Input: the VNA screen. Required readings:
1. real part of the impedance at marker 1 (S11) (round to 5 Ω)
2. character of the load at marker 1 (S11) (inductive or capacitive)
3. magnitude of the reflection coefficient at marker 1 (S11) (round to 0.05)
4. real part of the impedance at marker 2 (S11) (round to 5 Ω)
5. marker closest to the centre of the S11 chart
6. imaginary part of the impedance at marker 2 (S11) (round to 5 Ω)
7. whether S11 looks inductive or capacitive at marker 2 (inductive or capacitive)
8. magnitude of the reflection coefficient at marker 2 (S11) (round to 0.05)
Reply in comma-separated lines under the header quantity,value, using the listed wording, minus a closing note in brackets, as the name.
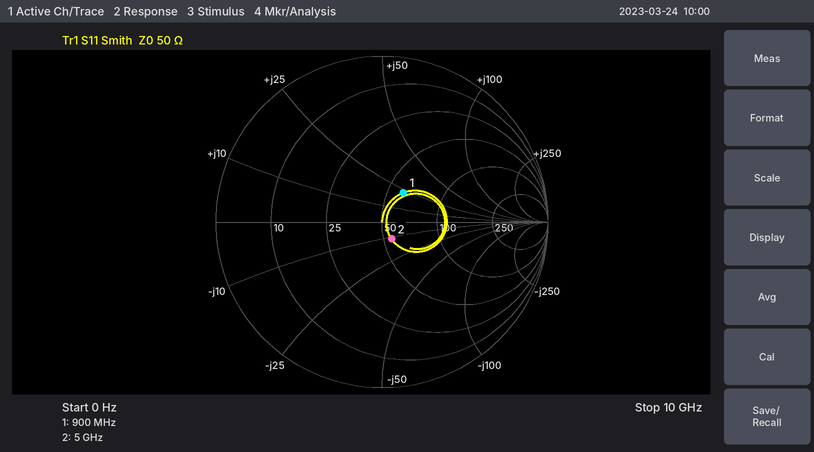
quantity,value
real part of the impedance at marker 1 (S11),60 Ω
character of the load at marker 1 (S11),inductive
magnitude of the reflection coefficient at marker 1 (S11),0.20
real part of the impedance at marker 2 (S11),55 Ω
marker closest to the centre of the S11 chart,marker 2
imaginary part of the impedance at marker 2 (S11),-10 Ω
whether S11 looks inductive or capacitive at marker 2,capacitive
magnitude of the reflection coefficient at marker 2 (S11),0.10
